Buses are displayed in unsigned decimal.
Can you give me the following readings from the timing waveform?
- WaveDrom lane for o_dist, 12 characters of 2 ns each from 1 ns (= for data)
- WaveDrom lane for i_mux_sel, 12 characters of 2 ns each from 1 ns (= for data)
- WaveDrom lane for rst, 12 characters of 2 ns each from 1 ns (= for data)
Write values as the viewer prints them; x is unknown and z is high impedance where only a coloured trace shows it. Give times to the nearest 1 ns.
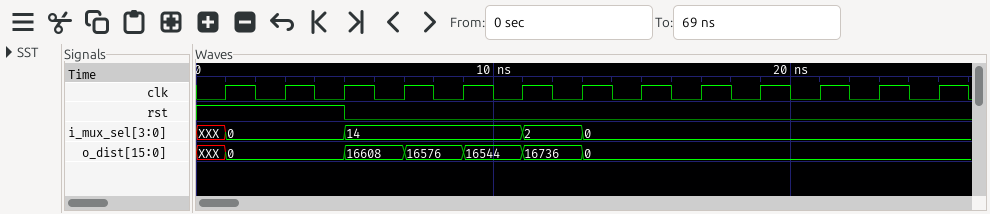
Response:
{name: 'o_dist', wave: '=.=====.....', data: '0 16608 16576 16544 16736 0'}
{name: 'i_mux_sel', wave: '=.=..==.....', data: '0 14 2 0'}
{name: 'rst', wave: '1.0.........'}
